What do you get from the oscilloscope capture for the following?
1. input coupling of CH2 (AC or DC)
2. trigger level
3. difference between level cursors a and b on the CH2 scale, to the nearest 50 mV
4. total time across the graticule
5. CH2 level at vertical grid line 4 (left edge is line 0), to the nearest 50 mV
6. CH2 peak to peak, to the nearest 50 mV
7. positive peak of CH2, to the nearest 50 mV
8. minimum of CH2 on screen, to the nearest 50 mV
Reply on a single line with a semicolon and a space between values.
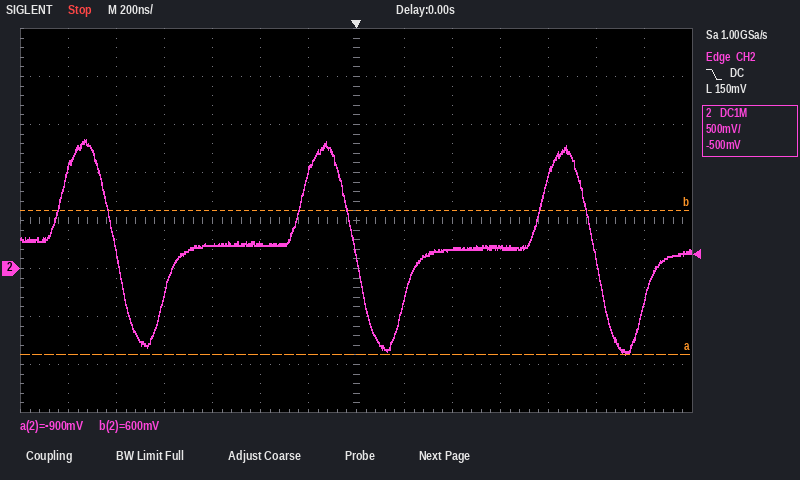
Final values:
DC; 150 mV; 1.50 V; 2.8 µs; 250 mV; 2.25 V; 1.35 V; -900 mV
